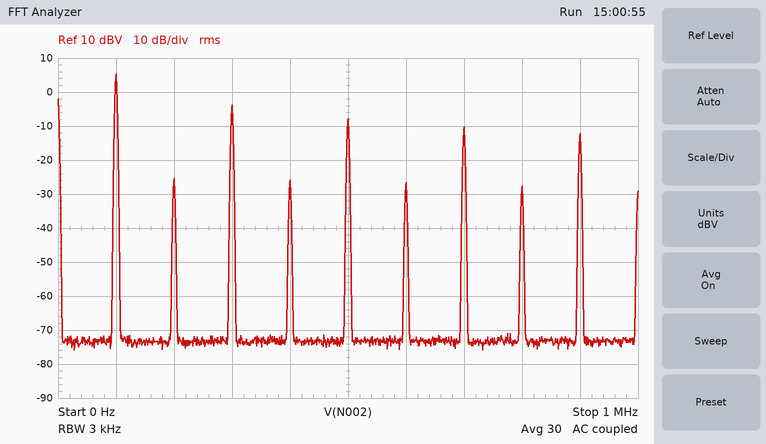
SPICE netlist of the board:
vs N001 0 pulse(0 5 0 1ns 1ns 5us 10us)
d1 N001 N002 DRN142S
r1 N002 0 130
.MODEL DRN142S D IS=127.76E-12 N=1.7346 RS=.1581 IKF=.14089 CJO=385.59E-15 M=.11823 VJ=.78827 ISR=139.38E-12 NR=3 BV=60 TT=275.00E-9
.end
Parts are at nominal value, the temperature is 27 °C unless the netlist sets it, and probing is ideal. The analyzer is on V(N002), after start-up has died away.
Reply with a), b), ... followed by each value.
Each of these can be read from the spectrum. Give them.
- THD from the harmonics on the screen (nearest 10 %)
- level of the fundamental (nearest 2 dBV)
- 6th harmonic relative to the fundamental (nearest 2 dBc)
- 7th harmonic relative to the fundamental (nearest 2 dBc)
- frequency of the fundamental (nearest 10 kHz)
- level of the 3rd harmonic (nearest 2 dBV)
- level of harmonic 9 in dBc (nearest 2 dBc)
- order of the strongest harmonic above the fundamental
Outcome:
a) 50 %
b) 6 dBV
c) -32 dBc
d) -16 dBc
e) 100 kHz
f) -4 dBV
g) -18 dBc
h) 3
